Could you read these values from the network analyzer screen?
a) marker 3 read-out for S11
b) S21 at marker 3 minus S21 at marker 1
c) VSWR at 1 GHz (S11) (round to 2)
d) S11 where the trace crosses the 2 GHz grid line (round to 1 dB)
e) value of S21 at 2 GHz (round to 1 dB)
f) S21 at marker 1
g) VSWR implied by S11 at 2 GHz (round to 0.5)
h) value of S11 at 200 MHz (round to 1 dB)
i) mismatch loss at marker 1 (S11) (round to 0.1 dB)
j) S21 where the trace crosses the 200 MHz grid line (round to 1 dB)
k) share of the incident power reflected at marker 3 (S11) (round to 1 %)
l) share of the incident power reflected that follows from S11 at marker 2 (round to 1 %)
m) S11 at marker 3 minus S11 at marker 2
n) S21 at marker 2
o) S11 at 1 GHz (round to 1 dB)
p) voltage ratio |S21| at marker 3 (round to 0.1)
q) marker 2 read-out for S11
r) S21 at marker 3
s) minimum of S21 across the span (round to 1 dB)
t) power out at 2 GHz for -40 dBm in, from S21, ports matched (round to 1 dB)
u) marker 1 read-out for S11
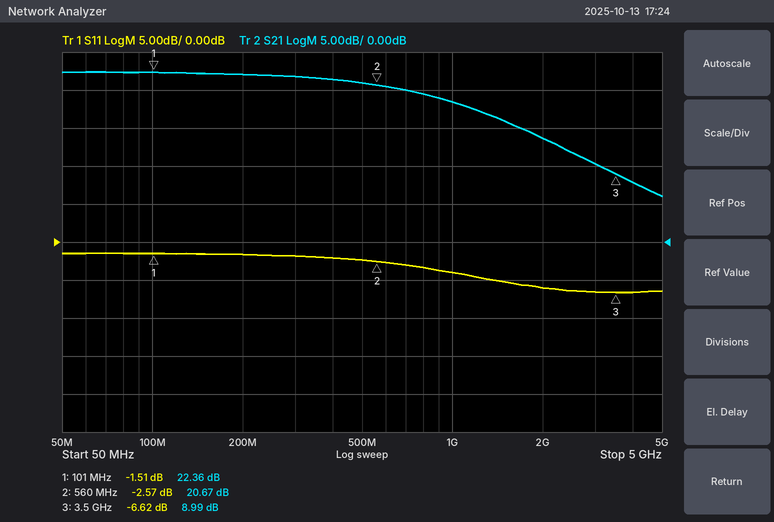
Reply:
-6.62 dB
-13.37 dB
4
-6 dB
14 dB
22.36 dB
3.0
-2 dB
5.3 dB
22 dB
22 %
55 %
-4.05 dB
20.67 dB
-4 dB
2.8
-2.57 dB
8.99 dB
6 dB
-26 dBm
-1.51 dB
